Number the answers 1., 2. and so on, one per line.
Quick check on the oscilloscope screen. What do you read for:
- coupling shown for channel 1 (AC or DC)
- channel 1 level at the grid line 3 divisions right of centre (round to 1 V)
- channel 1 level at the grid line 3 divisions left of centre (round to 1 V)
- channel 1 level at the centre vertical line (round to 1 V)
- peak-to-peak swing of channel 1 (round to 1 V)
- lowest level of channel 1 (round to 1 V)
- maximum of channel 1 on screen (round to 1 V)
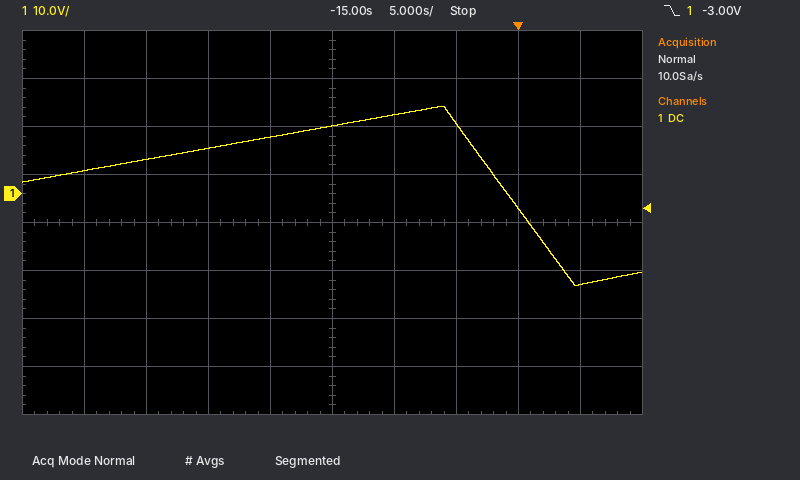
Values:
1. DC
2. -3 V
3. 7 V
4. 14 V
5. 37 V
6. -19 V
7. 18 V
